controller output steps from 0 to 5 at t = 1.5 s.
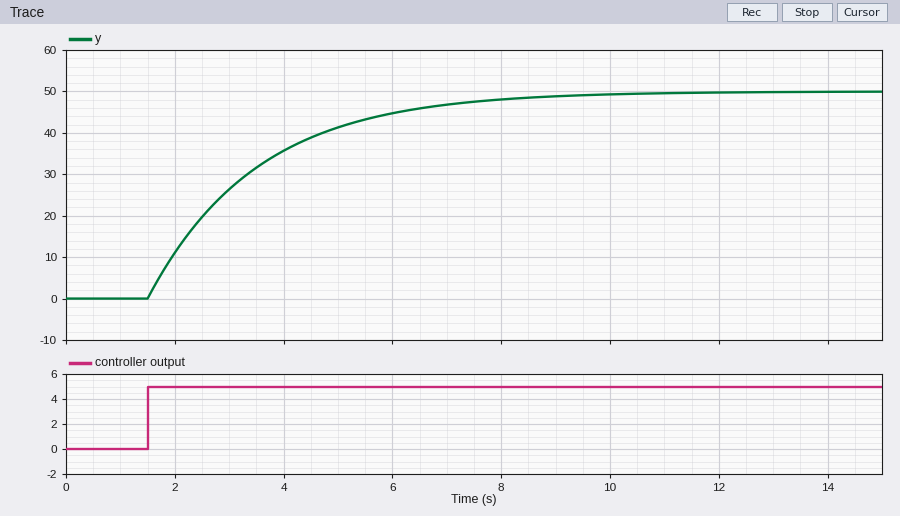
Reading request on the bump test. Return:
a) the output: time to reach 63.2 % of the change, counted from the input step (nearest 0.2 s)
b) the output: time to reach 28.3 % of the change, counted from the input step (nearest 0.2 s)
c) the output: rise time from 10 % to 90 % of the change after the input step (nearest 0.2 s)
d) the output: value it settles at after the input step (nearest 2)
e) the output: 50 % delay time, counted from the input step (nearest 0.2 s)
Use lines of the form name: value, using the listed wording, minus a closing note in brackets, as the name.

the output: time to reach 63.2 % of the change, counted from the input step: 2.0 s
the output: time to reach 28.3 % of the change, counted from the input step: 0.6 s
the output: rise time from 10 % to 90 % of the change after the input step: 4.4 s
the output: value it settles at after the input step: 50
the output: 50 % delay time, counted from the input step: 1.4 s
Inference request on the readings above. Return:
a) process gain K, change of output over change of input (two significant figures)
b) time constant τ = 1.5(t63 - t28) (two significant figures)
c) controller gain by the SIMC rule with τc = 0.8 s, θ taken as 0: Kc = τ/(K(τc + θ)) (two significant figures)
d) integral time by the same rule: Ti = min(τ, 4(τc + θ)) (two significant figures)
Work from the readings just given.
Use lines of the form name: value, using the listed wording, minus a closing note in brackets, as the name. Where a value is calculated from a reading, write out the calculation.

process gain K, change of output over change of input: (50 - 0) / 5 = 10
time constant τ = 1.5(t63 - t28): 1.5 × (2 - 0.6) = 2.1 s
controller gain by the SIMC rule with τc = 0.8 s, θ taken as 0: Kc = τ/(K(τc + θ)): 2.1 / (10 × (0.8 + 0)) = 0.26
integral time by the same rule: Ti = min(τ, 4(τc + θ)): min(2.1, 4 × (0.8 + 0)) = 2.1 s
